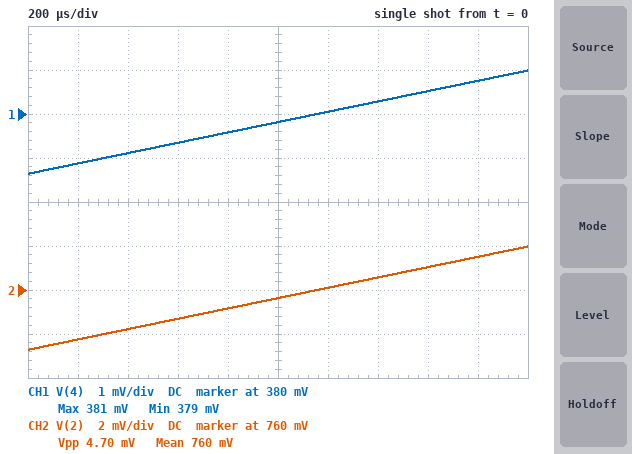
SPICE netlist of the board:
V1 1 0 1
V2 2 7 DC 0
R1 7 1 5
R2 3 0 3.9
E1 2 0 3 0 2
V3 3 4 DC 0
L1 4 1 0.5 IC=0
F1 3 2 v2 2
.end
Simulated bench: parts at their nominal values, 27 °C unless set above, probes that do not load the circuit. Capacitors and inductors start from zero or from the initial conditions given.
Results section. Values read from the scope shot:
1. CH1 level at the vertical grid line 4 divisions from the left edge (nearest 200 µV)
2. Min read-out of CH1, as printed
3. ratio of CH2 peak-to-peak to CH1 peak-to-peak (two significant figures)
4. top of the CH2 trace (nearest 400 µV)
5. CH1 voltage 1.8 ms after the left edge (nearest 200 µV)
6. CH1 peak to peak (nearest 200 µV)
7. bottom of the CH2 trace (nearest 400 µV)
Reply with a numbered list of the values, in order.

1. 379.6 mV
2. 379 mV
3. 2.0
4. 762.0 mV
5. 380.8 mV
6. 2.4 mV
7. 757.2 mV
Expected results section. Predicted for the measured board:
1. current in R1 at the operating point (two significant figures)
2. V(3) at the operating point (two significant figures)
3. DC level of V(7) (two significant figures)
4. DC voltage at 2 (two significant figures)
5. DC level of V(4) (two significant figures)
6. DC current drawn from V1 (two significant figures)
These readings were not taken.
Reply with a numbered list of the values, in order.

1. 200 mA
2. 1.0 V
3. 2.0 V
4. 2.0 V
5. 1.0 V
6. 460 mA
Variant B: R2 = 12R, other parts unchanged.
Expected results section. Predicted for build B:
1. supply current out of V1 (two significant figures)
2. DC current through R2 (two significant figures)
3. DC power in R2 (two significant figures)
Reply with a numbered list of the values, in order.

1. 280 mA
2. 83 mA
3. 83 mW
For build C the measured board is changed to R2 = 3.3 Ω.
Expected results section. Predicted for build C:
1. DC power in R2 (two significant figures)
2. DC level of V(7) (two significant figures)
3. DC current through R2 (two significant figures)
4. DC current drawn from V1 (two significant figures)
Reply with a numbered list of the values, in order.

1. 300 mW
2. 2.0 V
3. 300 mA
4. 500 mA
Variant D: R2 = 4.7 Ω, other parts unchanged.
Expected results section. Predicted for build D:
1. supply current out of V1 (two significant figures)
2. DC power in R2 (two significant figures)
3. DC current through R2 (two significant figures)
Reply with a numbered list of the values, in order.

1. 410 mA
2. 210 mW
3. 210 mA
